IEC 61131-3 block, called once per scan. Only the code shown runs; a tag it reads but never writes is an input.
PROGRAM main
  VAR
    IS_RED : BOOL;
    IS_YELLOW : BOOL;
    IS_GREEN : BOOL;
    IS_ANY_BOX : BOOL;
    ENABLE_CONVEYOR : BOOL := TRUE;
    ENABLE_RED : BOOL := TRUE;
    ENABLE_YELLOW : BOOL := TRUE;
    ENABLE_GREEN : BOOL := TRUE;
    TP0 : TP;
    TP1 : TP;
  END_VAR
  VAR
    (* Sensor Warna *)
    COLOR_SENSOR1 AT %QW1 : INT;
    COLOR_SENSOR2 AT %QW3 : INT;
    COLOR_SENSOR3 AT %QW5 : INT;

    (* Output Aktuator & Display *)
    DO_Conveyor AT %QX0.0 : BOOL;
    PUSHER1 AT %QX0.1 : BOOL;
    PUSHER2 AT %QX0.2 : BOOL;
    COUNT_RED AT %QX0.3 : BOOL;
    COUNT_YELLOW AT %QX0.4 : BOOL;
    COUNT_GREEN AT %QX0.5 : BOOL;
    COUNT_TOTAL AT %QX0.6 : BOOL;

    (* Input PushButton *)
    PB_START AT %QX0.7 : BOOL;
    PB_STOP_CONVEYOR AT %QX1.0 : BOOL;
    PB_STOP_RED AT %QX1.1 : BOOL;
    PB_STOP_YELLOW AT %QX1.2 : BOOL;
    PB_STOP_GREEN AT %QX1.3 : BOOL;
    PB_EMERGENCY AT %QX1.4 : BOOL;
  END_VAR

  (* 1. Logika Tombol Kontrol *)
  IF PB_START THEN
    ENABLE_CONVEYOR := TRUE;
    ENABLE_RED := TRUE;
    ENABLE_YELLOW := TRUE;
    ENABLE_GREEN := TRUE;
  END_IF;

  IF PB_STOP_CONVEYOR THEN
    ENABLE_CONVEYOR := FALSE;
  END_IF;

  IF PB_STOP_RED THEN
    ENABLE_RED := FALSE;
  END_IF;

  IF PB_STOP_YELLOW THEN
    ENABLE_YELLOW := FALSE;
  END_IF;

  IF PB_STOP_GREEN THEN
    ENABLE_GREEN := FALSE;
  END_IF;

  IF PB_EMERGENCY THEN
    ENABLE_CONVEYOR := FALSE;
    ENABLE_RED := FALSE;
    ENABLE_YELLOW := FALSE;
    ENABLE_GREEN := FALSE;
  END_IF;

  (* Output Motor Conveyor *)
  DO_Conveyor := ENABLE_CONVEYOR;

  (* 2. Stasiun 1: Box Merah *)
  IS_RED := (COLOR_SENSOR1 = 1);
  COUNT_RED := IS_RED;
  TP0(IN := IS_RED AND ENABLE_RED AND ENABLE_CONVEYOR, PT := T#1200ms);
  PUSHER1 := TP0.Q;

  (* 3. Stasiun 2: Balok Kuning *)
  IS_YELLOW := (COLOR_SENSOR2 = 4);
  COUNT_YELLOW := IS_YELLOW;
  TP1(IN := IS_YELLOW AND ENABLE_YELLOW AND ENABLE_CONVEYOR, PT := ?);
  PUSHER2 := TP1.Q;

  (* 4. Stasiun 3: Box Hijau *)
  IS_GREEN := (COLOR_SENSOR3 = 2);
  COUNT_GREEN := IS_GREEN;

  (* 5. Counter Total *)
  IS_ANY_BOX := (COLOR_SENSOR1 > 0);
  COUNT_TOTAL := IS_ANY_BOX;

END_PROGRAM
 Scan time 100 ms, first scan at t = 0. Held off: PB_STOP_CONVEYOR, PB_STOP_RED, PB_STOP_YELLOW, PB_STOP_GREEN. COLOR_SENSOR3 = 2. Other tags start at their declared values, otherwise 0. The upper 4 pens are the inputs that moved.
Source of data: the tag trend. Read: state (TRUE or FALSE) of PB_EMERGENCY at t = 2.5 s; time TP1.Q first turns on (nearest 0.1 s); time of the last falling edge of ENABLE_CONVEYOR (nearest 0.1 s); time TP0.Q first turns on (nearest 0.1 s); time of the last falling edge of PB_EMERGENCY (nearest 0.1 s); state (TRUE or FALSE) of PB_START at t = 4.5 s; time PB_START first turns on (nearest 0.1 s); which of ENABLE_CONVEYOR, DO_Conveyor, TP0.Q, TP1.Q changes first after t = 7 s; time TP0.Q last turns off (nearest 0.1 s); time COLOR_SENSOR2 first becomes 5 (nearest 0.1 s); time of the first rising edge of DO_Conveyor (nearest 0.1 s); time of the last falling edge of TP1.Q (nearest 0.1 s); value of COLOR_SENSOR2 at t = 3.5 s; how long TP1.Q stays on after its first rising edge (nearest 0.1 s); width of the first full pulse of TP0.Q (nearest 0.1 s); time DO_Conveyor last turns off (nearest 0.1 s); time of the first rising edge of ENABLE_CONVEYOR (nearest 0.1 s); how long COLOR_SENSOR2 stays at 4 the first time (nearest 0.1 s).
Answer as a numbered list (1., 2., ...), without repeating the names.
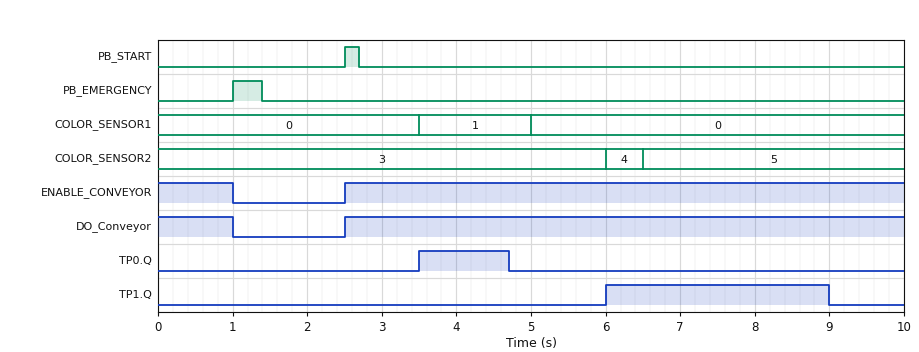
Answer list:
1. FALSE
2. 6.0 s
3. 1.0 s
4. 3.5 s
5. 1.4 s
6. FALSE
7. 2.5 s
8. TP1.Q
9. 4.7 s
10. 6.5 s
11. 2.5 s
12. 9.0 s
13. 3
14. 3.0 s
15. 1.2 s
16. 1.0 s
17. 2.5 s
18. 0.5 s
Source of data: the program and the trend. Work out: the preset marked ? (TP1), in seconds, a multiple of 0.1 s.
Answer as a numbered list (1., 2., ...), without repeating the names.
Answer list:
1. 3.0 s
